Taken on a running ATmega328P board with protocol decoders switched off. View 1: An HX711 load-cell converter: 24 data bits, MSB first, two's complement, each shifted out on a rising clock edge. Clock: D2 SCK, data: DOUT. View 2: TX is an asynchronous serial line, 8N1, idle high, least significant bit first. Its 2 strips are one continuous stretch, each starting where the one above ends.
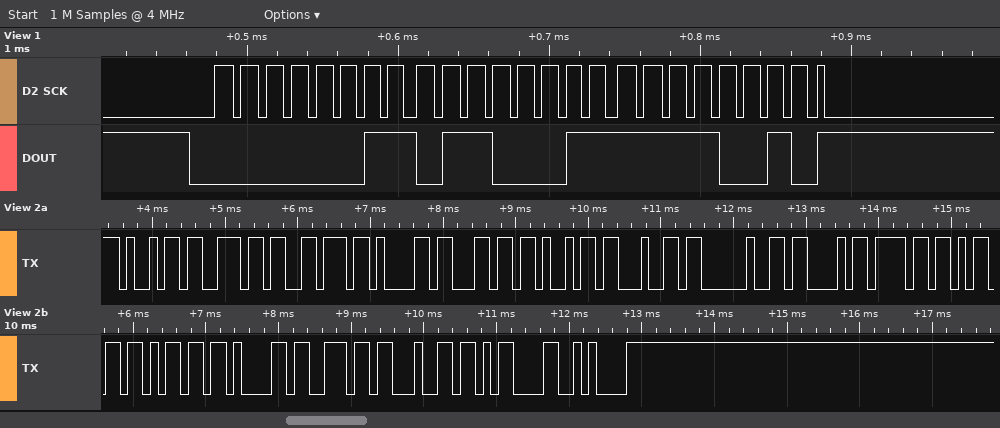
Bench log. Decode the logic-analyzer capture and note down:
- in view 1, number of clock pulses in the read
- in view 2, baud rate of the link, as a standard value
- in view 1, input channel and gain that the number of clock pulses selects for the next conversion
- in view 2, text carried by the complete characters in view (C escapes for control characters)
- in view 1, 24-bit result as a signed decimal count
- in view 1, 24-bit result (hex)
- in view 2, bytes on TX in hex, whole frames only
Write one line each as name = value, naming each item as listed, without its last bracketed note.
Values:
in view 1, number of clock pulses in the read = 25
in view 2, baud rate of the link, as a standard value = 9600 baud
in view 1, input channel and gain that the number of clock pulses selects for the next conversion = channel A, gain 128
in view 2, text carried by the complete characters in view = "invalid Command\r\n"
in view 1, 24-bit result as a signed decimal count = 222194
in view 1, 24-bit result = 0x0363F2
in view 2, bytes on TX in hex, whole frames only = 69 6E 76 61 6C 69 64 20 43 6F 6D 6D 61 6E 64 0D 0A
